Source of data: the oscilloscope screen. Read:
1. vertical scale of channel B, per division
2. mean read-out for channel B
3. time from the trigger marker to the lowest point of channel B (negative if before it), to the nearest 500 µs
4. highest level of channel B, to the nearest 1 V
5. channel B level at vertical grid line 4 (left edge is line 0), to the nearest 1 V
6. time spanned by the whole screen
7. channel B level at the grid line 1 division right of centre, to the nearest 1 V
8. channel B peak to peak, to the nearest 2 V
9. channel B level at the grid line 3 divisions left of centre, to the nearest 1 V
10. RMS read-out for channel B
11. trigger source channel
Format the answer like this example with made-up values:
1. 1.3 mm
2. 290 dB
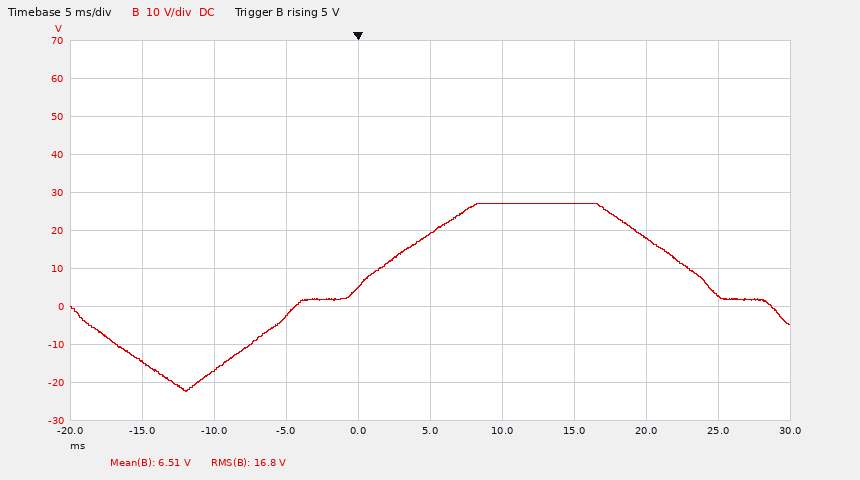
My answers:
1. 10 V
2. 6.51 V
3. -12.0 ms
4. 27 V
5. 5 V
6. 50 ms
7. 27 V
8. 50 V
9. -17 V
10. 16.8 V
11. channel B
